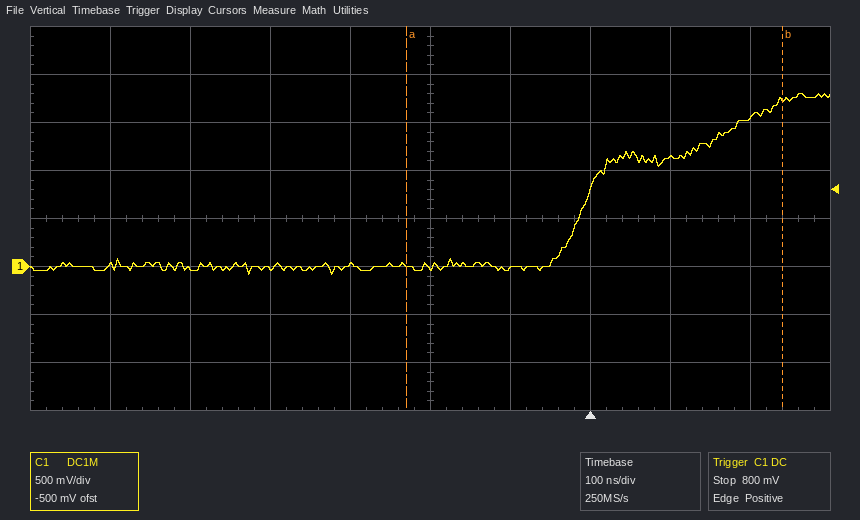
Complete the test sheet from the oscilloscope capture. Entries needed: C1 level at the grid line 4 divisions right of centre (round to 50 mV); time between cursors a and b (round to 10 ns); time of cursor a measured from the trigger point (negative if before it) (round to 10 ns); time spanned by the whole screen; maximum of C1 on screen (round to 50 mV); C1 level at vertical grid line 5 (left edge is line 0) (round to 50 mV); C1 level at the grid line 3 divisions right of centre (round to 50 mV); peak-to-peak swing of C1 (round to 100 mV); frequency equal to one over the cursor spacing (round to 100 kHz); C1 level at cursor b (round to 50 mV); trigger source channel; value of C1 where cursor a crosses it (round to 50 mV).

1.55 V
470 ns
-230 ns
1 µs
1.80 V
0 mV
1.15 V
1.90 V
2.1 MHz
1.75 V
C1
0 mV
